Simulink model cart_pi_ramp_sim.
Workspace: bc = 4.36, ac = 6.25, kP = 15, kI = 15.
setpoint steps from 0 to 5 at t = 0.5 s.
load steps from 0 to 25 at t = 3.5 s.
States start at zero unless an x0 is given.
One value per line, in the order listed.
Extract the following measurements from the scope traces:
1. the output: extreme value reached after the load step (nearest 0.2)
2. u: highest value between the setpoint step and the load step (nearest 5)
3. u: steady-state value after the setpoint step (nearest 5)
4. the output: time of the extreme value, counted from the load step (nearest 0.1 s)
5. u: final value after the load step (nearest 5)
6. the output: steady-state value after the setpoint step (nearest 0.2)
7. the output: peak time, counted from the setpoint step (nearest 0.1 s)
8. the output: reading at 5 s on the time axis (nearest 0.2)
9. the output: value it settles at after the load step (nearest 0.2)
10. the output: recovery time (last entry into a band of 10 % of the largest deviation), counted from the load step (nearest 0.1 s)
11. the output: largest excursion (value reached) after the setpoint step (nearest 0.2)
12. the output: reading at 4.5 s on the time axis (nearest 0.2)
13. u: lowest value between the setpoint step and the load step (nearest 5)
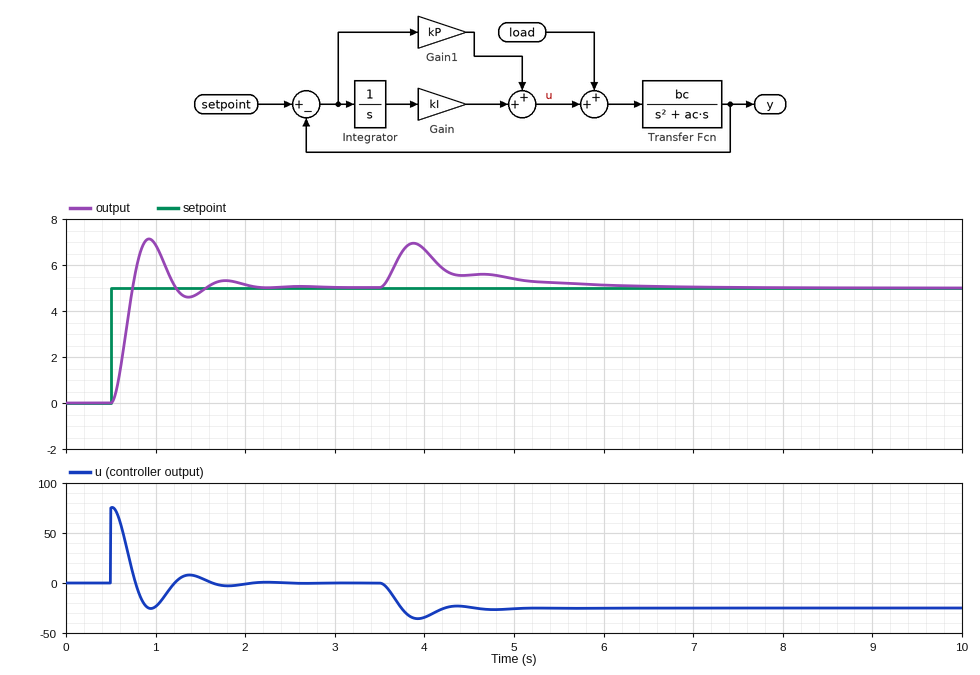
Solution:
7.0
75
0
0.4 s
-25
5.0
0.4 s
5.4
5.0
2.2 s
7.2
5.6
-25
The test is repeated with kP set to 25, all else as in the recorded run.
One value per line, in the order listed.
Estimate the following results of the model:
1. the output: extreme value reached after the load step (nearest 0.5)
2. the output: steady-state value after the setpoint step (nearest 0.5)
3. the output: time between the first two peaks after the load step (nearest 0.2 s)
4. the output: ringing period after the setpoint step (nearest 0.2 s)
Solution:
6.5
5.0
0.6 s
0.6 s
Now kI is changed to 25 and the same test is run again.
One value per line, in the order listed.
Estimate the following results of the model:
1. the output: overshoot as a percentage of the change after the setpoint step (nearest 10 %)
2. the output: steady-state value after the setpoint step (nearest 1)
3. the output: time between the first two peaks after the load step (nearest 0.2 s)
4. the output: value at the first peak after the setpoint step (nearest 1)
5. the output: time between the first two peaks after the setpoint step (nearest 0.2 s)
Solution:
50 %
5
0.8 s
8
0.8 s
